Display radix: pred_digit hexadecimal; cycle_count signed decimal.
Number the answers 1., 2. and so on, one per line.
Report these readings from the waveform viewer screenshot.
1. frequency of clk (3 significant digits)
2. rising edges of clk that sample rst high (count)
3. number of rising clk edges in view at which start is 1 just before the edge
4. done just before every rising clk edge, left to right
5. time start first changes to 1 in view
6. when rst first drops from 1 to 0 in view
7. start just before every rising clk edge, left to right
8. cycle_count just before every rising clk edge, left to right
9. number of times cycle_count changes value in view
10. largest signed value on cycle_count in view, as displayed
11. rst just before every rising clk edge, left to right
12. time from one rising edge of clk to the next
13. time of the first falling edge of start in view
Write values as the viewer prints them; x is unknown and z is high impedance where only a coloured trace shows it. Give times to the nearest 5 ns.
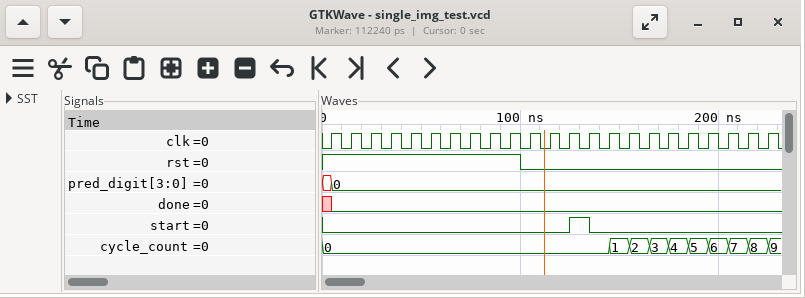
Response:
1. 100 MHz
2. 10
3. 1
4. x 0 0 0 0 0 0 0 0 0 0 0 0 0 0 0 0 0 0 0 0 0 0
5. 125 ns
6. 100 ns
7. 0 0 0 0 0 0 0 0 0 0 0 0 0 1 0 0 0 0 0 0 0 0 0
8. 0, 0, 0, 0, 0, 0, 0, 0, 0, 0, 0, 0, 0, 0, 0, 1, 2, 3, 4, 5, 6, 7, 8
9. 9
10. 9
11. 1 1 1 1 1 1 1 1 1 1 0 0 0 0 0 0 0 0 0 0 0 0 0
12. 10 ns
13. 135 ns
